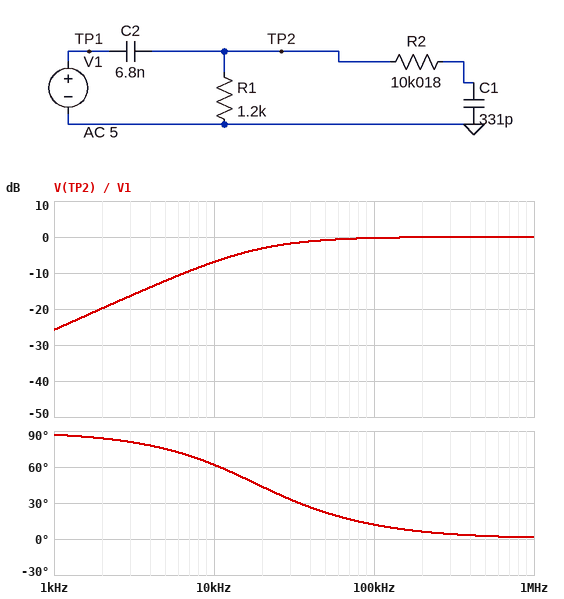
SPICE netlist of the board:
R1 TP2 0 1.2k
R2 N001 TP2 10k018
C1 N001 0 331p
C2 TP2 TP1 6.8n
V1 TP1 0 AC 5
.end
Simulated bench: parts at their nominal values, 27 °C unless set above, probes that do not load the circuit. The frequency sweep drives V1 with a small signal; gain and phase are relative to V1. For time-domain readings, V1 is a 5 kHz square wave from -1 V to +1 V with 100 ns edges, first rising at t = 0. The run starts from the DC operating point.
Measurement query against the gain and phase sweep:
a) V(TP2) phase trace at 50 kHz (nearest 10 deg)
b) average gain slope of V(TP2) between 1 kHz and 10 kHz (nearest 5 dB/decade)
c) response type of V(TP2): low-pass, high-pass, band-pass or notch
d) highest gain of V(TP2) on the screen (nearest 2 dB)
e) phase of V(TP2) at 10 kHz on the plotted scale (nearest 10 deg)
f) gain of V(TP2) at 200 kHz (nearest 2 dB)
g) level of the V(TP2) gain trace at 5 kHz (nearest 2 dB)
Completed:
20 deg
20 dB/decade
high-pass
0 dB
60 deg
0 dB
-12 dB
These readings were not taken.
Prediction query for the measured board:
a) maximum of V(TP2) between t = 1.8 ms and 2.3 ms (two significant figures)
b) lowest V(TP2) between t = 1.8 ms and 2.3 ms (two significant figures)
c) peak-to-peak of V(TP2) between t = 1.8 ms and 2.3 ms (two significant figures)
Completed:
2.0 V
-2.0 V
4.0 V
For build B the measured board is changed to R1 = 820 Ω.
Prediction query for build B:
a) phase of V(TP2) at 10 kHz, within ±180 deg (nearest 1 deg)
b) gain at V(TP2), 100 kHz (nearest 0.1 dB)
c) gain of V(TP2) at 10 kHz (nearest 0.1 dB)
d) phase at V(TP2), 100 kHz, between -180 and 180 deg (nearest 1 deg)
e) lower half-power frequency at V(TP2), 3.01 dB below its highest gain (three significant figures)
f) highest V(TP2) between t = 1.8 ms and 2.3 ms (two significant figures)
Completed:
70 deg
-0.5 dB
-9.7 dB
17 deg
30.3 kHz
2.0 V
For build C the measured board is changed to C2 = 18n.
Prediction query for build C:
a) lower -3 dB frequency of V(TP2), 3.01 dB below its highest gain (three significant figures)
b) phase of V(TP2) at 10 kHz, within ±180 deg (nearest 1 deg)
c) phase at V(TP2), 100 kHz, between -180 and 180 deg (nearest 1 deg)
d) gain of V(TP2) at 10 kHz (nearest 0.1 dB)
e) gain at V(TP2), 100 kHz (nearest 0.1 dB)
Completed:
7.53 kHz
36 deg
5 deg
-2.0 dB
-0.1 dB
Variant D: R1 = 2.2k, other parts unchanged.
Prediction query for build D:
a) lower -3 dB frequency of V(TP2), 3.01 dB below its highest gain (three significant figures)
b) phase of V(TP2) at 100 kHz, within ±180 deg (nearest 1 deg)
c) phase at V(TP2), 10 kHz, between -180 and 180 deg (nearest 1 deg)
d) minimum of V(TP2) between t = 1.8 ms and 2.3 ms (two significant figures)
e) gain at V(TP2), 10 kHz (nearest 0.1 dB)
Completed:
11.3 kHz
7 deg
46 deg
-2.0 V
-3.5 dB
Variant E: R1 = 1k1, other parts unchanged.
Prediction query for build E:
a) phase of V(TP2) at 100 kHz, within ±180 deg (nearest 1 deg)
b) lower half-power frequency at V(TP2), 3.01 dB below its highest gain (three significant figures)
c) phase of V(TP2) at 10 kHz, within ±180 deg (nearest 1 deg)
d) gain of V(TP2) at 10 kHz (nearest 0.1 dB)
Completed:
13 deg
22.6 kHz
64 deg
-7.5 dB
